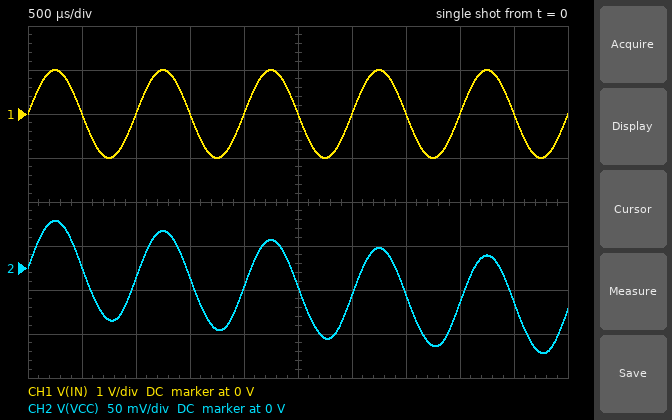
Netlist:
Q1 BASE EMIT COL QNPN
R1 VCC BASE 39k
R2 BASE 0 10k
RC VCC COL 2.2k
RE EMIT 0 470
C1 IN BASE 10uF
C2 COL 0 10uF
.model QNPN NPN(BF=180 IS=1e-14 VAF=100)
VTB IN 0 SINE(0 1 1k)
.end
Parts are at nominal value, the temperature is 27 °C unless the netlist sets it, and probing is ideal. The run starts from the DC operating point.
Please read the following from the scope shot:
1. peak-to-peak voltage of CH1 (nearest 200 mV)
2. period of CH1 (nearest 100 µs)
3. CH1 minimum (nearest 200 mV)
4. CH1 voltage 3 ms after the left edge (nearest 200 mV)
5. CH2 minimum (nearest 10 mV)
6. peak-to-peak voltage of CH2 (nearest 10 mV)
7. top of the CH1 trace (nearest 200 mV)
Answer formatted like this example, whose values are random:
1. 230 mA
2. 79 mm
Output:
1. 2.0 V
2. 1.0 ms
3. -1.0 V
4. 0 V
5. -100 mV
6. 150 mV
7. 1.0 V
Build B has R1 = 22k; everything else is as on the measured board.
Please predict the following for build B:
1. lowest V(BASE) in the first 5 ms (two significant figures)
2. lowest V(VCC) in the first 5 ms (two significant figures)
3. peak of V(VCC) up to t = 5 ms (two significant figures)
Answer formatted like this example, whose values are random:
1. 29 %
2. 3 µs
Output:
1. -990 mV
2. -130 mV
3. 91 mV
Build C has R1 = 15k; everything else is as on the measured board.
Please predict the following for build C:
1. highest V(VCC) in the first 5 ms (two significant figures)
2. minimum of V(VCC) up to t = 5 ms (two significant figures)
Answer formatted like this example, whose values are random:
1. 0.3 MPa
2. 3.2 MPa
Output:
1. 130 mV
2. -160 mV
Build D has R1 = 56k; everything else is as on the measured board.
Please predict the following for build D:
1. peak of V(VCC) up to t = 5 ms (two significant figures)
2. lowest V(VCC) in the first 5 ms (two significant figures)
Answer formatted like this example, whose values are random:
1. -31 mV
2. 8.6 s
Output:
1. 38 mV
2. -84 mV
